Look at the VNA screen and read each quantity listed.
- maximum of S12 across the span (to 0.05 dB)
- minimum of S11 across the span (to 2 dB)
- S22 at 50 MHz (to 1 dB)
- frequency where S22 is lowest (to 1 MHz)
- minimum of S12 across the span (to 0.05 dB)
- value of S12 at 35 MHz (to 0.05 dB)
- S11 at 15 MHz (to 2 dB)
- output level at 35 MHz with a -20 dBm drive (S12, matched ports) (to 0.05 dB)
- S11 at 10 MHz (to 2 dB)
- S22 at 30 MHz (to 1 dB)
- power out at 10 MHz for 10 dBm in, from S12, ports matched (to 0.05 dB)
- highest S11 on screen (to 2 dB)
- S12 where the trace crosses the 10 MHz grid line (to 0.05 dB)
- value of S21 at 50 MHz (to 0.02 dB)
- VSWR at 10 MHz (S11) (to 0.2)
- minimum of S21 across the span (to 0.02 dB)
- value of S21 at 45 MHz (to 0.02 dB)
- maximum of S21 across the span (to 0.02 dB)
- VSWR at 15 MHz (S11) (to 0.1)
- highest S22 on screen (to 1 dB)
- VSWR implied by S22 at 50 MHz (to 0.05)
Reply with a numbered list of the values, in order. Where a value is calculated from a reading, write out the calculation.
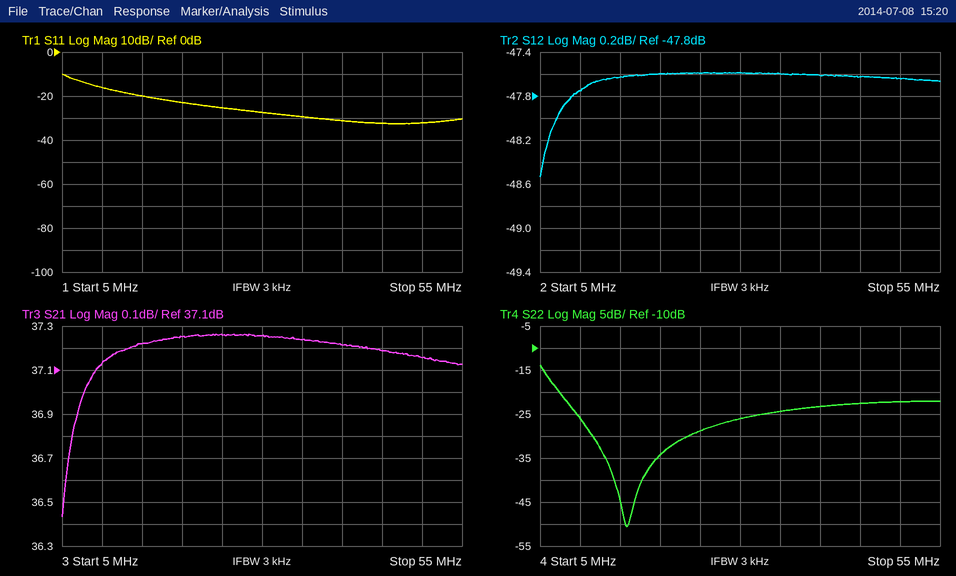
1. -47.60 dB
2. -32 dB
3. -22 dB
4. 16 MHz
5. -48.55 dB
6. -47.60 dB
7. -20 dB
8. -20 dBm + (-47.60 dB) = -67.60 dBm
9. -16 dB
10. -26 dB
11. 10 dBm + (-47.75 dB) = -37.75 dBm
12. -10 dB
13. -47.75 dB
14. 37.16 dB
15. |Γ| = 10^(-16/20) = 0.1585; VSWR = (1 + 0.1585)/(1 − 0.1585) ≈ 1.4
16. 36.44 dB
17. 37.18 dB
18. 37.26 dB
19. |Γ| = 10^(-20/20) = 0.1000; VSWR = (1 + 0.1000)/(1 − 0.1000) ≈ 1.2
20. -14 dB
21. |Γ| = 10^(-22/20) = 0.0794; VSWR = (1 + 0.0794)/(1 − 0.0794) ≈ 1.17, so 1.15 to the nearest 0.05
